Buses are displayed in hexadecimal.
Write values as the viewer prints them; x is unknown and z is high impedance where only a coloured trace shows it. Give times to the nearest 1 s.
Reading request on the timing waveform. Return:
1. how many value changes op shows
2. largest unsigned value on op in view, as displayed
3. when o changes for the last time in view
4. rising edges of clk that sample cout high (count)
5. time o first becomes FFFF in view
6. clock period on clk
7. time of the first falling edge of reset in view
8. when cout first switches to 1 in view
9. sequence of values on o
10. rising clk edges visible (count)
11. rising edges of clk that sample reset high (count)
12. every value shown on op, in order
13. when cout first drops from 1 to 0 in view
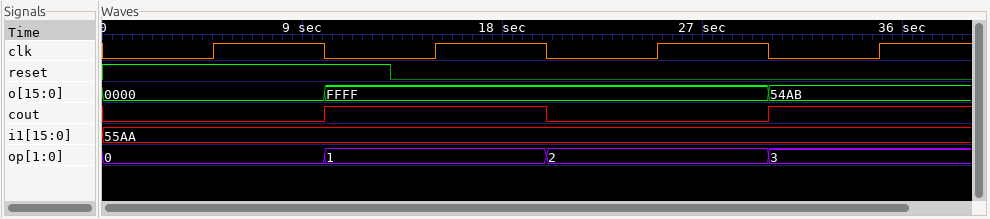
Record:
3
3
30 s
2
10 s
10 s
13 s
10 s
0000, FFFF, 54AB
4
1
0, 1, 2, 3
20 s
